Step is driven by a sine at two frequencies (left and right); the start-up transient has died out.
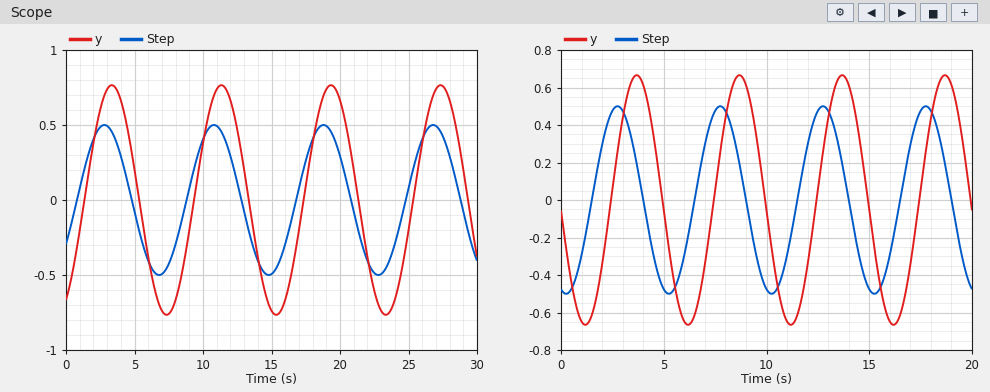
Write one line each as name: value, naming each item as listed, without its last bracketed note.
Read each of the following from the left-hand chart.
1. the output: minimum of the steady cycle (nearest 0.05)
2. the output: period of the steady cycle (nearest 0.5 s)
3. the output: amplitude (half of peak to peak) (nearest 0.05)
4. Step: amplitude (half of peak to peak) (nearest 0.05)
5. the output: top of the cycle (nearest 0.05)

the output: minimum of the steady cycle: -0.75
the output: period of the steady cycle: 8.0 s
the output: amplitude (half of peak to peak): 0.75
Step: amplitude (half of peak to peak): 0.50
the output: top of the cycle: 0.75
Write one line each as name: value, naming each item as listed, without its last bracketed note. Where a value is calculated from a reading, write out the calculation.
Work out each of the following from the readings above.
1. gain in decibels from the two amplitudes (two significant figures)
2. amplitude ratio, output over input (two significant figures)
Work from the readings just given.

gain in decibels from the two amplitudes: 20 log10(0.75 / 0.5) = 3.5 dB
amplitude ratio, output over input: 0.75 / 0.5 = 1.5
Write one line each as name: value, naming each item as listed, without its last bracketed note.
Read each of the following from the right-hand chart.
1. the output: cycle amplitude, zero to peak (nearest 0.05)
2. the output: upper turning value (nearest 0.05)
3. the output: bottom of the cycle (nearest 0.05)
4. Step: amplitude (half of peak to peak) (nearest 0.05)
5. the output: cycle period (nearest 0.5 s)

the output: cycle amplitude, zero to peak: 0.65
the output: upper turning value: 0.65
the output: bottom of the cycle: -0.65
Step: amplitude (half of peak to peak): 0.50
the output: cycle period: 5.0 s
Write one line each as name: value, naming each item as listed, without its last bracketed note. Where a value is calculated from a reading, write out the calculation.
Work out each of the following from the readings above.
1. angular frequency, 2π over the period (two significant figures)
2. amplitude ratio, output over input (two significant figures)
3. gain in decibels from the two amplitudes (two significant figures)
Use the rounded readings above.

angular frequency, 2π over the period: 2π / 5 = 1.3 rad/s
amplitude ratio, output over input: 0.65 / 0.5 = 1.3
gain in decibels from the two amplitudes: 20 log10(0.65 / 0.5) = 2.3 dB
